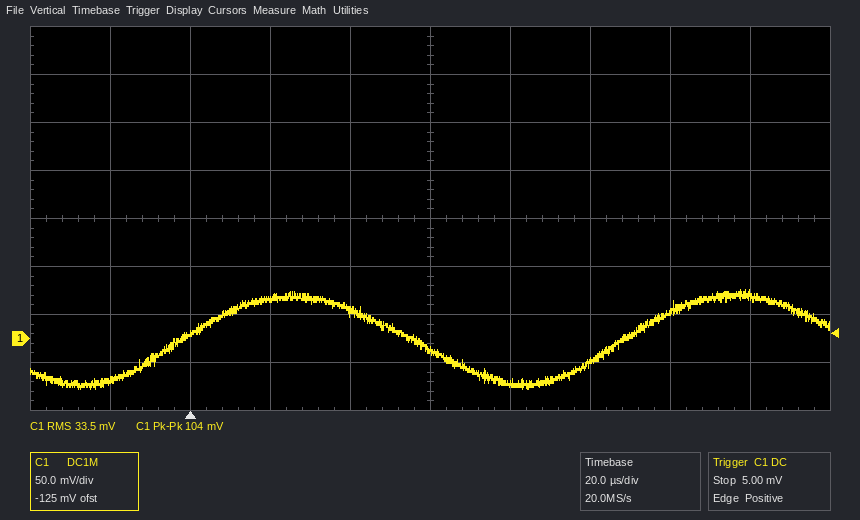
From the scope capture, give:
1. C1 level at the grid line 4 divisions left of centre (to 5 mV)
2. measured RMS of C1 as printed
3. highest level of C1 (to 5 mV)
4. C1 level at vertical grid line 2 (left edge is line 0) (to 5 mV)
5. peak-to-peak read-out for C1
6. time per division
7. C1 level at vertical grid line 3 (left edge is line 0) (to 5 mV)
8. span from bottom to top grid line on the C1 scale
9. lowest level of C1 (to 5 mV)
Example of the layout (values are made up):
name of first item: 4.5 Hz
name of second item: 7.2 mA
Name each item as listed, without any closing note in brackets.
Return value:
C1 level at the grid line 4 divisions left of centre: -45 mV
measured RMS of C1 as printed: 33.5 mV
highest level of C1: 50 mV
C1 level at vertical grid line 2 (left edge is line 0): 5 mV
peak-to-peak read-out for C1: 104 mV
time per division: 20 µs
C1 level at vertical grid line 3 (left edge is line 0): 40 mV
span from bottom to top grid line on the C1 scale: 400 mV
lowest level of C1: -55 mV
